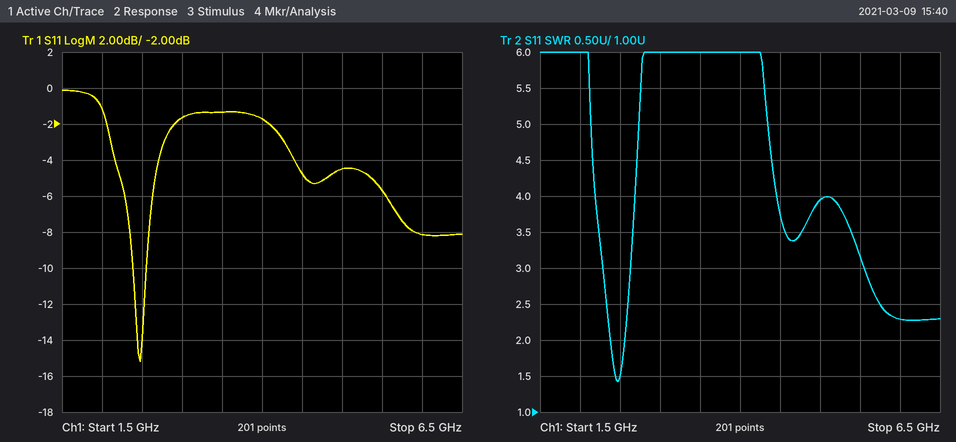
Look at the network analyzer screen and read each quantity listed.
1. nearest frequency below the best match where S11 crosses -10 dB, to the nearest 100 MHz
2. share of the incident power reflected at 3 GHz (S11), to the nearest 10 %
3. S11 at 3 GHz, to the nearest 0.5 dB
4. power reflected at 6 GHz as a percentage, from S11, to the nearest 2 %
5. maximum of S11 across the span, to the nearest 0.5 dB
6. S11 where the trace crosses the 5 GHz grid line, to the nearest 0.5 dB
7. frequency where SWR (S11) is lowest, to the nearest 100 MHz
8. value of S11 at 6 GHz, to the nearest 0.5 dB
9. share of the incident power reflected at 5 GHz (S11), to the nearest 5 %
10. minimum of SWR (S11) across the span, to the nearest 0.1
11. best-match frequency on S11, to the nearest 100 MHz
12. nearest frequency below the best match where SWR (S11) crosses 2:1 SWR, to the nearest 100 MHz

2.4 GHz
70 %
-1.5 dB
16 %
0.0 dB
-4.5 dB
2.5 GHz
-8.0 dB
35 %
1.4
2.5 GHz
2.4 GHz
